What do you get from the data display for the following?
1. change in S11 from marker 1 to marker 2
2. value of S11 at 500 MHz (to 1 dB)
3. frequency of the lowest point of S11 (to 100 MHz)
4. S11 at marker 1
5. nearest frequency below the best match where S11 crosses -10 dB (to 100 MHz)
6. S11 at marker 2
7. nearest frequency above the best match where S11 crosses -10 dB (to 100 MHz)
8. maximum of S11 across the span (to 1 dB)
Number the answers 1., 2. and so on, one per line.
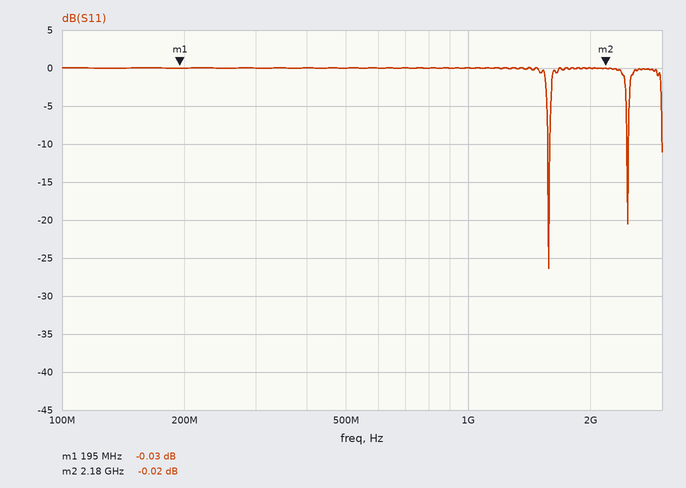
1. 0.01 dB
2. 0 dB
3. 1.6 GHz
4. -0.03 dB
5. 1.6 GHz
6. -0.02 dB
7. 1.6 GHz
8. 0 dB
